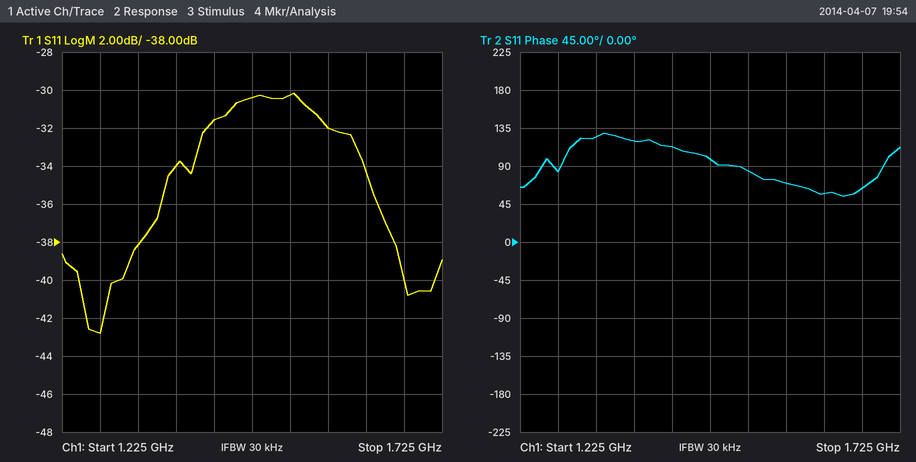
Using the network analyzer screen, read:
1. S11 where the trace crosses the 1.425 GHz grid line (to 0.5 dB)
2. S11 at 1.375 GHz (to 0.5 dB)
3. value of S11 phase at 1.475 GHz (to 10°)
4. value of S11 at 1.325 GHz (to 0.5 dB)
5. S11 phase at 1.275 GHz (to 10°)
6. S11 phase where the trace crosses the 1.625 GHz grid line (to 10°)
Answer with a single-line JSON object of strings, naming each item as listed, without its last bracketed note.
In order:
{"S11 where the trace crosses the 1.425 GHz grid line": "-31.5 dB", "S11 at 1.375 GHz": "-34.0 dB", "value of S11 phase at 1.475 GHz": "100°", "value of S11 at 1.325 GHz": "-38.0 dB", "S11 phase at 1.275 GHz": "80°", "S11 phase where the trace crosses the 1.625 GHz grid line": "60°"}
